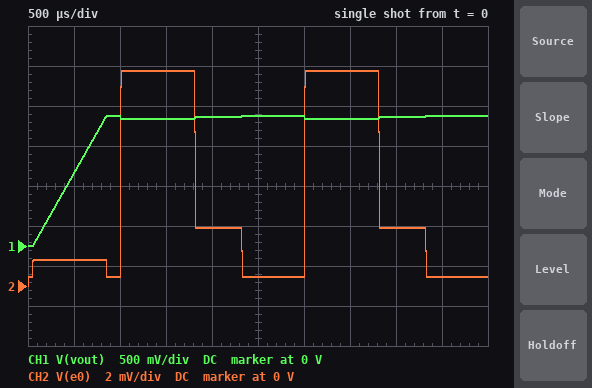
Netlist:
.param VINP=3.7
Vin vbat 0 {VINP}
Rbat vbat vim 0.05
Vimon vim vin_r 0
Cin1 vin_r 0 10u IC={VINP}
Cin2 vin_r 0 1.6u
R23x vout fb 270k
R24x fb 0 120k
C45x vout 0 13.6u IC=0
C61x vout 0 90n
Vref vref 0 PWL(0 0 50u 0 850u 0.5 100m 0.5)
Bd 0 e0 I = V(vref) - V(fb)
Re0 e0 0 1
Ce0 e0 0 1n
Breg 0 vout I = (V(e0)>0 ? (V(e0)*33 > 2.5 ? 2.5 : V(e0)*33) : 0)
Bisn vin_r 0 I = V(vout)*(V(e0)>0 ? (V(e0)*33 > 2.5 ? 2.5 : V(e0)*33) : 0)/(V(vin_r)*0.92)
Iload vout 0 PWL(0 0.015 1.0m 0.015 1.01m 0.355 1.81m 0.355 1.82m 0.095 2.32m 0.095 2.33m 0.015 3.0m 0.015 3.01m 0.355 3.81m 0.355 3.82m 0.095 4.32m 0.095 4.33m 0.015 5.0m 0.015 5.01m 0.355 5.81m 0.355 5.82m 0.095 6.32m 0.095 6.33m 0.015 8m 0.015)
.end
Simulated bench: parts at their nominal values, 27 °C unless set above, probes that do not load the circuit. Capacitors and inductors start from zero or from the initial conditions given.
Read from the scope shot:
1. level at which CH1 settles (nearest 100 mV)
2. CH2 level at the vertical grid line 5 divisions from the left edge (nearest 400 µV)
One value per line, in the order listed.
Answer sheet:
1.6 V
400 µV
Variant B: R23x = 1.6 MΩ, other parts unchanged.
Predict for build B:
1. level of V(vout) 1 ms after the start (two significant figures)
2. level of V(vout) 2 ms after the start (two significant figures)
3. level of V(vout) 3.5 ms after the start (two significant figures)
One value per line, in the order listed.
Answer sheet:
7.2 V
7.1 V
7.0 V
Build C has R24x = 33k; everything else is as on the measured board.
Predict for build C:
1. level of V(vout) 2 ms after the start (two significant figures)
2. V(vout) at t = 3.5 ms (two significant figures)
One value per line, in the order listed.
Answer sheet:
4.6 V
4.5 V
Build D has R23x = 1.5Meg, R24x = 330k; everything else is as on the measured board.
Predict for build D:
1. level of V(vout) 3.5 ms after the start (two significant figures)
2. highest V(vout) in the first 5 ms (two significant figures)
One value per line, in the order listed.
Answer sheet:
2.7 V
2.8 V
